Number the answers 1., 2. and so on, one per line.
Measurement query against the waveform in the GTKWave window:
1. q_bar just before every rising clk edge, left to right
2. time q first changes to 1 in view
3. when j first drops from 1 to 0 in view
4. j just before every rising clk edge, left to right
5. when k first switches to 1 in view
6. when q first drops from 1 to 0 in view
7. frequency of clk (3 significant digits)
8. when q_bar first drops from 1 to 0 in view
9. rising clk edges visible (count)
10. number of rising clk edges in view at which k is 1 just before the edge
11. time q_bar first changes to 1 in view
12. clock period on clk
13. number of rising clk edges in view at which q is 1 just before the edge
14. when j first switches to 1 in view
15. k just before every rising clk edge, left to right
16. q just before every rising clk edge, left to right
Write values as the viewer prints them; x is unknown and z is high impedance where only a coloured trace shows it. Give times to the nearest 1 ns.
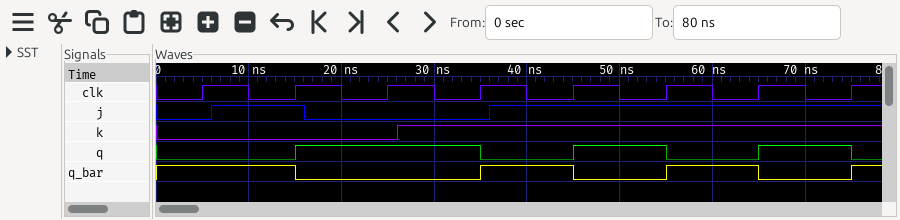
1. 1 1 0 0 1 0 1 0
2. 15 ns
3. 16 ns
4. 0 1 0 0 1 1 1 1
5. 26 ns
6. 35 ns
7. 100 MHz
8. 15 ns
9. 8
10. 5
11. 35 ns
12. 10 ns
13. 4
14. 6 ns
15. 0 0 0 1 1 1 1 1
16. 0 0 1 1 0 1 0 1
